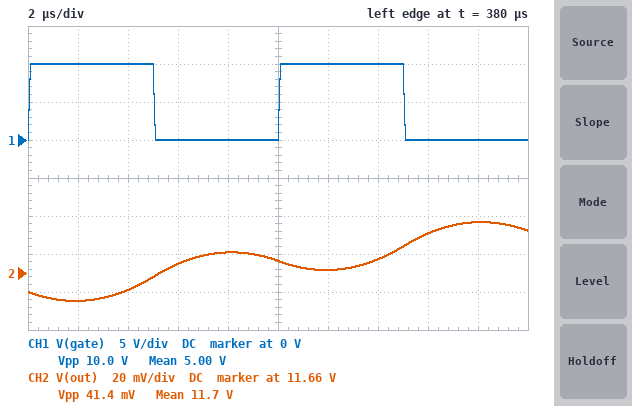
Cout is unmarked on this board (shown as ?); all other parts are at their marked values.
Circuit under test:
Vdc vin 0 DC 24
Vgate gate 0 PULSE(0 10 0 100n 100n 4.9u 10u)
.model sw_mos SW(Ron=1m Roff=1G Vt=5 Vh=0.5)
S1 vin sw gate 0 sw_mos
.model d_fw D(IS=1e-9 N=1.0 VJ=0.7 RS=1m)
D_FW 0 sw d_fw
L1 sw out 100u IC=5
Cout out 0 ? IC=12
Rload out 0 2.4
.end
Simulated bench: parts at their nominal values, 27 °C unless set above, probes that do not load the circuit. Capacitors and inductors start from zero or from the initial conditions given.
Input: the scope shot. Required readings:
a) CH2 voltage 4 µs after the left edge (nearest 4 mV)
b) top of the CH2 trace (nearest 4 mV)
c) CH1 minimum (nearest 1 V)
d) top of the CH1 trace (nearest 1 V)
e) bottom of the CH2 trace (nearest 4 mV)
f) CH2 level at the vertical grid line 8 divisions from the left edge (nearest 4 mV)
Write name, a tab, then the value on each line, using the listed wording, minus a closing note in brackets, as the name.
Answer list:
CH2 voltage 4 µs after the left edge	11.652 V
top of the CH2 trace	11.688 V
CH1 minimum	0 V
top of the CH1 trace	10 V
bottom of the CH2 trace	11.644 V
CH2 level at the vertical grid line 8 divisions from the left edge	11.680 V
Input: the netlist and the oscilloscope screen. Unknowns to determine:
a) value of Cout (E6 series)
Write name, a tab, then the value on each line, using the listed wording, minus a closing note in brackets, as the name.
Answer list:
value of Cout	47 µF
